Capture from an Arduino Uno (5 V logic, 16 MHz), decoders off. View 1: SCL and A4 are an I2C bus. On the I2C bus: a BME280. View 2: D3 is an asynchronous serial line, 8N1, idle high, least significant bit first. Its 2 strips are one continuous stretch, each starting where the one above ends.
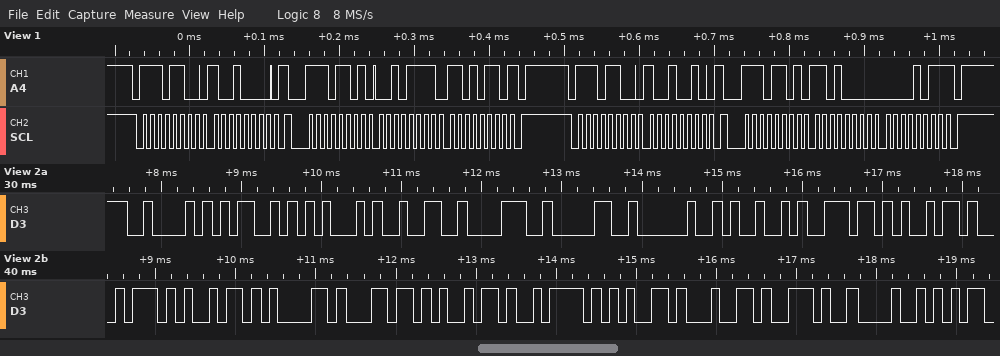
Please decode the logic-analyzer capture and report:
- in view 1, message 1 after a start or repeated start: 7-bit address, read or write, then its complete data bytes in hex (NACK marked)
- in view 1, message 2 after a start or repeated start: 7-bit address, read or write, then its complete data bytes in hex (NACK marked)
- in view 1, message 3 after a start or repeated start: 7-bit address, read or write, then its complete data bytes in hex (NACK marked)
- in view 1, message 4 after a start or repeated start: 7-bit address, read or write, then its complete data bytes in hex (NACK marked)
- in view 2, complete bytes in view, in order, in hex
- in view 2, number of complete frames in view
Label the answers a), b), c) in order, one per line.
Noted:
a) 0x76 write: 90
b) 0x76 read: 2F D6 NACK
c) 0x76 write: 92
d) 0x76 read: D0 0B NACK
e) 42 4D 45 32 38 30 20 49 6E 69 74 69 61 6C 69 7A 65 64 2E 48
f) 20
